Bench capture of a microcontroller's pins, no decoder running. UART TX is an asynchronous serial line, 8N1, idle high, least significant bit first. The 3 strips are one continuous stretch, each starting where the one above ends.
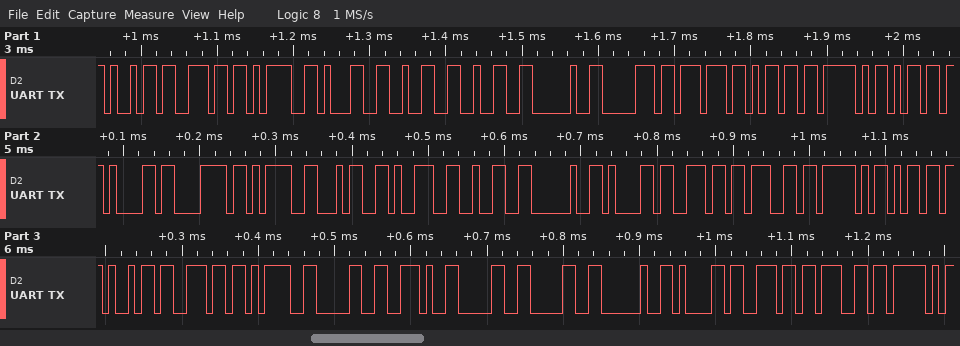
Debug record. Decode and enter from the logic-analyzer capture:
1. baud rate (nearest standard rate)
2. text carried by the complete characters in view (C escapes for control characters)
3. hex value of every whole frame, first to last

115200 baud
"in=122 pwm_max=492 ang_min=0.00 ang_"
69 6E 3D 31 32 32 20 70 77 6D 5F 6D 61 78 3D 34 39 32 20 61 6E 67 5F 6D 69 6E 3D 30 2E 30 30 20 61 6E 67 5F
